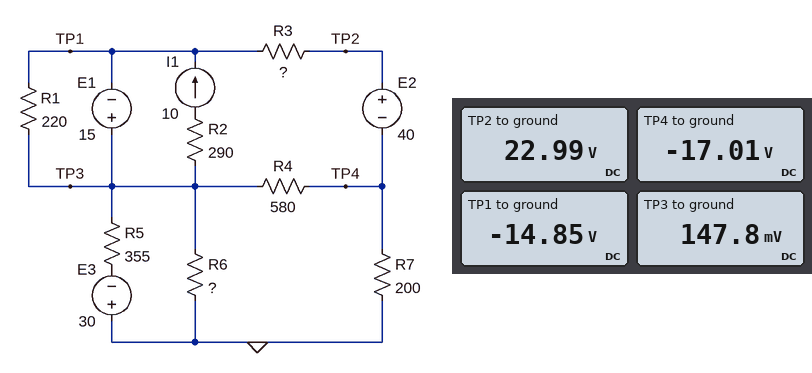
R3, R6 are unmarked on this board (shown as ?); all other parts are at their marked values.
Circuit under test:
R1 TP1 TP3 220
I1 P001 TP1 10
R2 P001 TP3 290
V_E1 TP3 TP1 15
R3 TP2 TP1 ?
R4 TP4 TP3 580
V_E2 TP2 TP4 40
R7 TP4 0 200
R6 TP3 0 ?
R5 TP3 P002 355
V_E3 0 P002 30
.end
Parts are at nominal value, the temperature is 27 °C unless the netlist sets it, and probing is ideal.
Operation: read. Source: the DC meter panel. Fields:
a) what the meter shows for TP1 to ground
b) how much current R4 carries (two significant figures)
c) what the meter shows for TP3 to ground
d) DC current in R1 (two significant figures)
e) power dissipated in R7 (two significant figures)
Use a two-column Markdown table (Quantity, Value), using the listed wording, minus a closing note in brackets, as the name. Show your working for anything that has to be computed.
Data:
| Quantity | Value |
|---|---|
| what the meter shows for TP1 to ground | -14.85 V |
| how much current R4 carries | (147.8 mV - (-17.01 V)) / 580 Ω = 30 mA |
| what the meter shows for TP3 to ground | 147.8 mV |
| DC current in R1 | (147.8 mV - (-14.85 V)) / 220 Ω = 68 mA |
| power dissipated in R7 | (0 V - (-17.01 V))^2 / 200 Ω = 1.4 W |
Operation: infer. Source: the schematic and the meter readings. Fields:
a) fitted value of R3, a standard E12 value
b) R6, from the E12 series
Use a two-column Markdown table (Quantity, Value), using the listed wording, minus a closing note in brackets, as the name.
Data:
| Quantity | Value |
|---|---|
| fitted value of R3, a standard E12 value | 330 Ω |
| R6, from the E12 series | 1 kΩ |
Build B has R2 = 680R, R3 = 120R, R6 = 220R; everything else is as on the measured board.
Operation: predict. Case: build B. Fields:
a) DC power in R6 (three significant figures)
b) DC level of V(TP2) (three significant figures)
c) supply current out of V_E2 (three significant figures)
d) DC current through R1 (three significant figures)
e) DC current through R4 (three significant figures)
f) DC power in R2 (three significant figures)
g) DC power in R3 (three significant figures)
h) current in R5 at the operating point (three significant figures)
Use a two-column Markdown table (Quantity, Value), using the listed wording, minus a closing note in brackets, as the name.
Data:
| Quantity | Value |
|---|---|
| DC power in R6 | 182 mW |
| DC level of V(TP2) | 13.8 V |
| supply current out of V_E2 | 187 mA |
| DC current through R1 | 68.2 mA |
| DC current through R4 | 56.1 mA |
| DC power in R2 | 68.0 kW |
| DC power in R3 | 4.20 W |
| current in R5 at the operating point | 102 mA |
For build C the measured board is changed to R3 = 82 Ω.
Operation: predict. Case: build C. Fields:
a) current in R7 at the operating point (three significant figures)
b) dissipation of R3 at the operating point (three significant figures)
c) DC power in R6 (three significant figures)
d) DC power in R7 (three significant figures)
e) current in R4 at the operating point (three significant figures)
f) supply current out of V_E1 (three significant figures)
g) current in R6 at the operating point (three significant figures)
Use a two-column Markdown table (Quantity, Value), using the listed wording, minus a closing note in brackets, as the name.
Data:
| Quantity | Value |
|---|---|
| current in R7 at the operating point | 132 mA |
| dissipation of R3 at the operating point | 3.23 W |
| DC power in R6 | 153 mW |
| DC power in R7 | 3.47 W |
| current in R4 at the operating point | 66.8 mA |
| supply current out of V_E1 | 10.3 A |
| current in R6 at the operating point | 12.4 mA |
